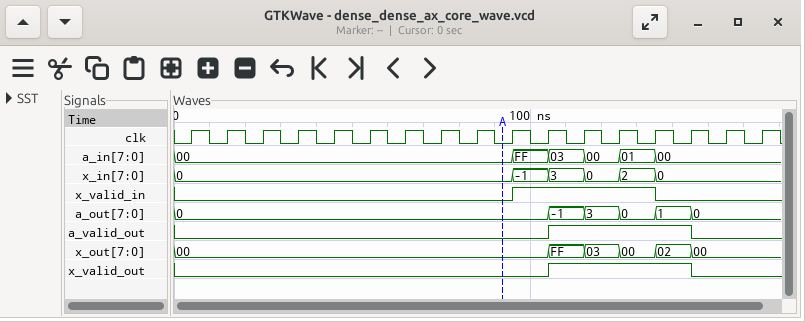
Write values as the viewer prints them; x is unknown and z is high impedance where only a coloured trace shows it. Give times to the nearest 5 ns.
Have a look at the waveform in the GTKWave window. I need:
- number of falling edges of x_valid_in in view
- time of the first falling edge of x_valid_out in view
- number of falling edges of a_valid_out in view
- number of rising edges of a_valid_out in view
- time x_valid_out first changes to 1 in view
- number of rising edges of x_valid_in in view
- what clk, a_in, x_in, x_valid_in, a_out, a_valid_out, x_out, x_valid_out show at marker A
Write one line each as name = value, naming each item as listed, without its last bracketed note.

number of falling edges of x_valid_in in view = 1
time of the first falling edge of x_valid_out in view = 145 ns
number of falling edges of a_valid_out in view = 1
number of rising edges of a_valid_out in view = 1
time x_valid_out first changes to 1 in view = 105 ns
number of rising edges of x_valid_in in view = 1
what clk, a_in, x_in, x_valid_in, a_out, a_valid_out, x_out, x_valid_out show at marker A = clk=0, a_in=00, x_in=0, x_valid_in=0, a_out=0, a_valid_out=0, x_out=00, x_valid_out=0
